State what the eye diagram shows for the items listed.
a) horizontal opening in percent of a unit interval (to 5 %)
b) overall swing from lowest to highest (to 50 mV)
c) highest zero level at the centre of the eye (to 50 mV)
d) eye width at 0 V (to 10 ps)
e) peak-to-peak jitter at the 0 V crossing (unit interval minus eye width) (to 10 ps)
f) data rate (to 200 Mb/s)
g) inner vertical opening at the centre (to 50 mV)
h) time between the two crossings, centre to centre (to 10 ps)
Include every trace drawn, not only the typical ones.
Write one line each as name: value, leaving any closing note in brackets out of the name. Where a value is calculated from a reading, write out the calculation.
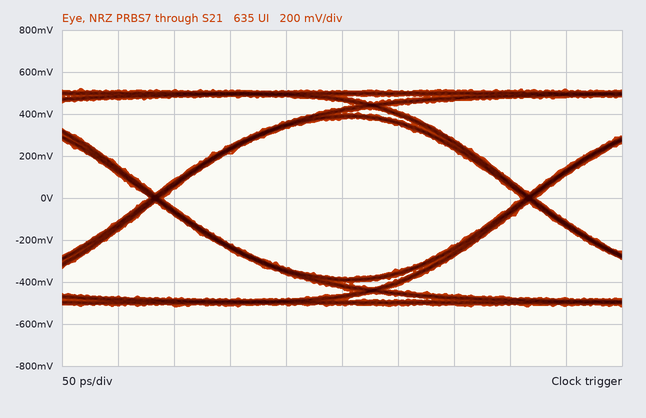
horizontal opening in percent of a unit interval: 320 ps / 330 ps ≈ 97.0 %, so 95 % to the nearest 5 %
overall swing from lowest to highest: 1.05 V
highest zero level at the centre of the eye: -400 mV
eye width at 0 V: 320 ps
peak-to-peak jitter at the 0 V crossing (unit interval minus eye width): 10 ps
data rate: 3.0 Gb/s
inner vertical opening at the centre: 750 mV
time between the two crossings, centre to centre: 330 ps
